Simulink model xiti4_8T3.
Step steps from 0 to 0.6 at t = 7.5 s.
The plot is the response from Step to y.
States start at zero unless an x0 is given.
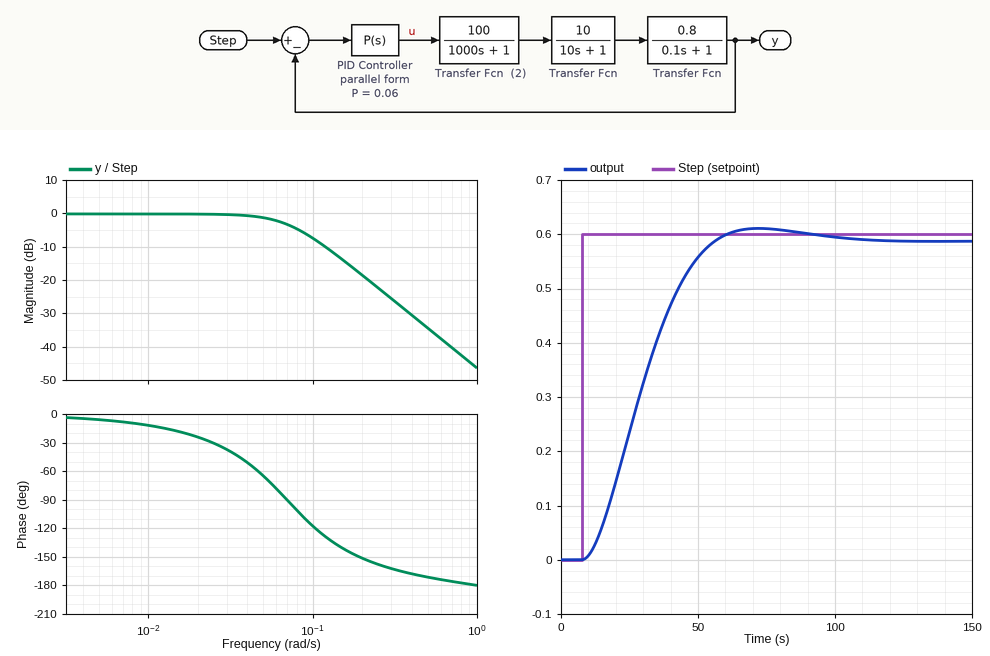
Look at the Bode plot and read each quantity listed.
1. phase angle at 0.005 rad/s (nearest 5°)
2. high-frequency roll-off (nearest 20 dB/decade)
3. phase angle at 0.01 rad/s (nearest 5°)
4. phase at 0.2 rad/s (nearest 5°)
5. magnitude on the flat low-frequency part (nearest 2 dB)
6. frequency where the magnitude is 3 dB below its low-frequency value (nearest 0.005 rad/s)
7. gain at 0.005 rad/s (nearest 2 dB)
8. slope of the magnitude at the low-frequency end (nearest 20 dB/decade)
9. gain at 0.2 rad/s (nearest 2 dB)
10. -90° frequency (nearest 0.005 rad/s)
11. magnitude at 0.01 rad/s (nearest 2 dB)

-5°
-40 dB/decade
-10°
-150°
0 dB
0.070 rad/s
0 dB
0 dB/decade
-18 dB
0.070 rad/s
0 dB
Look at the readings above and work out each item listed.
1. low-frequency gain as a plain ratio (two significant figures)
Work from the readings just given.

1.0
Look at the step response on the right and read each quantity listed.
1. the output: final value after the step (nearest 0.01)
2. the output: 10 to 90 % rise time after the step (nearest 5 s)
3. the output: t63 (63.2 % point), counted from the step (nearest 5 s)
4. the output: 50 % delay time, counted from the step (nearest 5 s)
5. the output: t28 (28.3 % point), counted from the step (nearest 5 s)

0.59
30 s
25 s
20 s
15 s
